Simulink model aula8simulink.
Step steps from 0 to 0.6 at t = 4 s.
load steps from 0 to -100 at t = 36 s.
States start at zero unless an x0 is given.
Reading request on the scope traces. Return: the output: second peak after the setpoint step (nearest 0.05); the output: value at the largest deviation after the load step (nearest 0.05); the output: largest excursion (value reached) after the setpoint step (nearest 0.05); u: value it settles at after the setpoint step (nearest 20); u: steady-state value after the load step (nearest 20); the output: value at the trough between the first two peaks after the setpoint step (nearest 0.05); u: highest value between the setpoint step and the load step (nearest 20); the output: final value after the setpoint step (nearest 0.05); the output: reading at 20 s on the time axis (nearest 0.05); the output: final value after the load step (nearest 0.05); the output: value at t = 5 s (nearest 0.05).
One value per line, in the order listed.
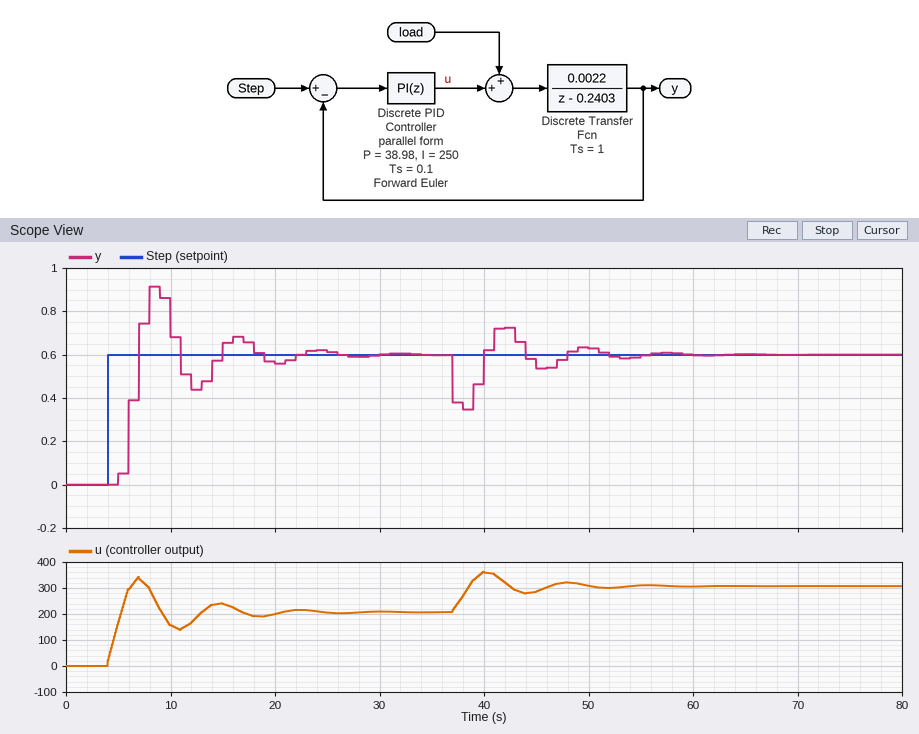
0.70
0.35
0.90
200
300
0.45
340
0.60
0.55
0.60
0.05
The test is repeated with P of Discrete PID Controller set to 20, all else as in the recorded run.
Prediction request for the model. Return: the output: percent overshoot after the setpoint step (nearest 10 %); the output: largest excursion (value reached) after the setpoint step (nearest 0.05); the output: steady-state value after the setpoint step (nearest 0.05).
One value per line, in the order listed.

60 %
0.95
0.60
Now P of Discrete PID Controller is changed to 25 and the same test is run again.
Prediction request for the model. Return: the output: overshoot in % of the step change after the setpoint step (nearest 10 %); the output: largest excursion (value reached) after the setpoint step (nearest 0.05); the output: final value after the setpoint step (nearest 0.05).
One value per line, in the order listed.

60 %
0.95
0.60
